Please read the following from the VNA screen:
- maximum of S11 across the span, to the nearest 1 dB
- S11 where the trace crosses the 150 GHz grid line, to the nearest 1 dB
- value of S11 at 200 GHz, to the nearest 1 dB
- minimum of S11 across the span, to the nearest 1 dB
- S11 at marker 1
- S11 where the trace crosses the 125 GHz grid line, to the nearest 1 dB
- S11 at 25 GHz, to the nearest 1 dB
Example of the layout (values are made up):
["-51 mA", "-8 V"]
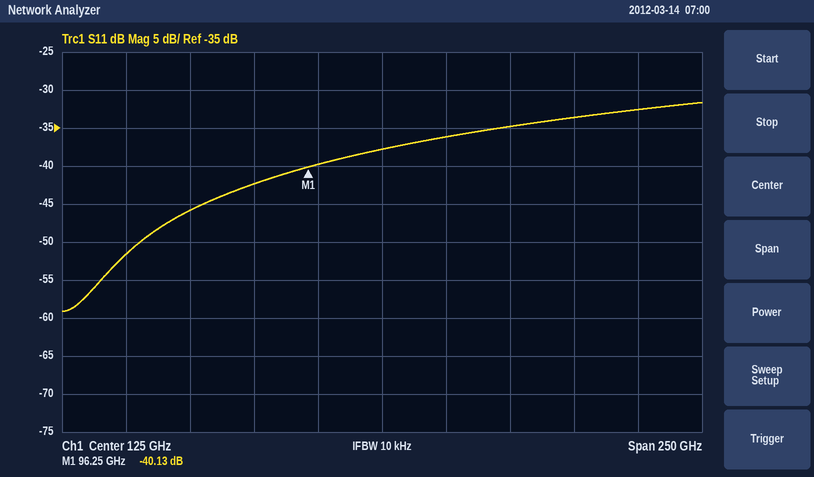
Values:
["-32 dB", "-36 dB", "-34 dB", "-59 dB", "-40.13 dB", "-38 dB", "-52 dB"]
